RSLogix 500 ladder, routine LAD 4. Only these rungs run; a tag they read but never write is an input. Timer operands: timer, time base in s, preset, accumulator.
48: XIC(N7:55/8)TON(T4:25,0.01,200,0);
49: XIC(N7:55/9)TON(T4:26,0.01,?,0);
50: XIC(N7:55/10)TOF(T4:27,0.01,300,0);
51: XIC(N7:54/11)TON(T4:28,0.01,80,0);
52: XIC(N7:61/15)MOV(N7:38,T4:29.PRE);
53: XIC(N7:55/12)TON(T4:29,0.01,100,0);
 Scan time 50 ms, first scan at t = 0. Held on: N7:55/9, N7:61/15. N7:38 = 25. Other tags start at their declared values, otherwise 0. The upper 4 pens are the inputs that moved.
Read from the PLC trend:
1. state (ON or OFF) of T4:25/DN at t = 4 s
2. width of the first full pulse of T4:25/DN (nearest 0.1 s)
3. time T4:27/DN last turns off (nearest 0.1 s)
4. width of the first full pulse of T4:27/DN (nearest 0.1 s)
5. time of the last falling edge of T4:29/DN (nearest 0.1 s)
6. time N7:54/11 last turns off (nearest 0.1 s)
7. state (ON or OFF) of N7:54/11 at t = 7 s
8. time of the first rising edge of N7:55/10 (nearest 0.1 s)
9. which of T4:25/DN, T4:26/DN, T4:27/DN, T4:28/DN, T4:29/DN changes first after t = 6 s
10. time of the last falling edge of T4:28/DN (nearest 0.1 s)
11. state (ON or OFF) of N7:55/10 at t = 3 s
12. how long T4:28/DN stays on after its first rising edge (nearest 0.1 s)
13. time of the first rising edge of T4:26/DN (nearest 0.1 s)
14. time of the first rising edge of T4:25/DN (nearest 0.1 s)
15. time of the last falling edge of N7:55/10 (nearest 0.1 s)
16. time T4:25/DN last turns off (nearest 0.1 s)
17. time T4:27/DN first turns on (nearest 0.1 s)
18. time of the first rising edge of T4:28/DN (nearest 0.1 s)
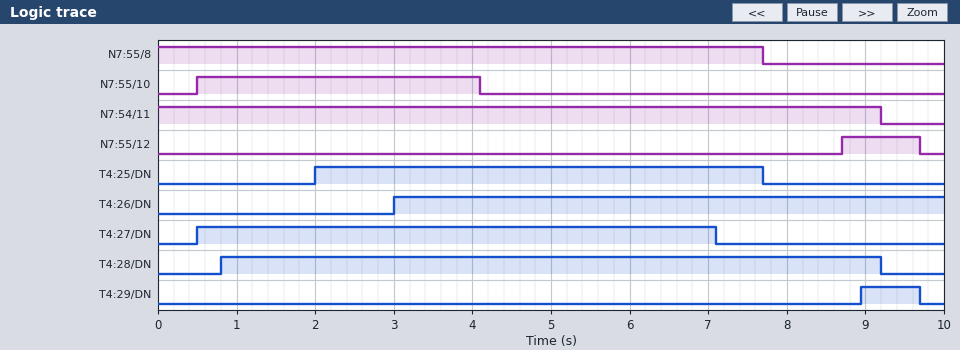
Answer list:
ON
5.7 s
7.1 s
6.6 s
9.7 s
9.2 s
ON
0.5 s
T4:27/DN
9.2 s
ON
8.4 s
3.0 s
2.0 s
4.1 s
7.7 s
0.5 s
0.8 s
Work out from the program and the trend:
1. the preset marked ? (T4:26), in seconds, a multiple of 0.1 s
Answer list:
3.0 s
